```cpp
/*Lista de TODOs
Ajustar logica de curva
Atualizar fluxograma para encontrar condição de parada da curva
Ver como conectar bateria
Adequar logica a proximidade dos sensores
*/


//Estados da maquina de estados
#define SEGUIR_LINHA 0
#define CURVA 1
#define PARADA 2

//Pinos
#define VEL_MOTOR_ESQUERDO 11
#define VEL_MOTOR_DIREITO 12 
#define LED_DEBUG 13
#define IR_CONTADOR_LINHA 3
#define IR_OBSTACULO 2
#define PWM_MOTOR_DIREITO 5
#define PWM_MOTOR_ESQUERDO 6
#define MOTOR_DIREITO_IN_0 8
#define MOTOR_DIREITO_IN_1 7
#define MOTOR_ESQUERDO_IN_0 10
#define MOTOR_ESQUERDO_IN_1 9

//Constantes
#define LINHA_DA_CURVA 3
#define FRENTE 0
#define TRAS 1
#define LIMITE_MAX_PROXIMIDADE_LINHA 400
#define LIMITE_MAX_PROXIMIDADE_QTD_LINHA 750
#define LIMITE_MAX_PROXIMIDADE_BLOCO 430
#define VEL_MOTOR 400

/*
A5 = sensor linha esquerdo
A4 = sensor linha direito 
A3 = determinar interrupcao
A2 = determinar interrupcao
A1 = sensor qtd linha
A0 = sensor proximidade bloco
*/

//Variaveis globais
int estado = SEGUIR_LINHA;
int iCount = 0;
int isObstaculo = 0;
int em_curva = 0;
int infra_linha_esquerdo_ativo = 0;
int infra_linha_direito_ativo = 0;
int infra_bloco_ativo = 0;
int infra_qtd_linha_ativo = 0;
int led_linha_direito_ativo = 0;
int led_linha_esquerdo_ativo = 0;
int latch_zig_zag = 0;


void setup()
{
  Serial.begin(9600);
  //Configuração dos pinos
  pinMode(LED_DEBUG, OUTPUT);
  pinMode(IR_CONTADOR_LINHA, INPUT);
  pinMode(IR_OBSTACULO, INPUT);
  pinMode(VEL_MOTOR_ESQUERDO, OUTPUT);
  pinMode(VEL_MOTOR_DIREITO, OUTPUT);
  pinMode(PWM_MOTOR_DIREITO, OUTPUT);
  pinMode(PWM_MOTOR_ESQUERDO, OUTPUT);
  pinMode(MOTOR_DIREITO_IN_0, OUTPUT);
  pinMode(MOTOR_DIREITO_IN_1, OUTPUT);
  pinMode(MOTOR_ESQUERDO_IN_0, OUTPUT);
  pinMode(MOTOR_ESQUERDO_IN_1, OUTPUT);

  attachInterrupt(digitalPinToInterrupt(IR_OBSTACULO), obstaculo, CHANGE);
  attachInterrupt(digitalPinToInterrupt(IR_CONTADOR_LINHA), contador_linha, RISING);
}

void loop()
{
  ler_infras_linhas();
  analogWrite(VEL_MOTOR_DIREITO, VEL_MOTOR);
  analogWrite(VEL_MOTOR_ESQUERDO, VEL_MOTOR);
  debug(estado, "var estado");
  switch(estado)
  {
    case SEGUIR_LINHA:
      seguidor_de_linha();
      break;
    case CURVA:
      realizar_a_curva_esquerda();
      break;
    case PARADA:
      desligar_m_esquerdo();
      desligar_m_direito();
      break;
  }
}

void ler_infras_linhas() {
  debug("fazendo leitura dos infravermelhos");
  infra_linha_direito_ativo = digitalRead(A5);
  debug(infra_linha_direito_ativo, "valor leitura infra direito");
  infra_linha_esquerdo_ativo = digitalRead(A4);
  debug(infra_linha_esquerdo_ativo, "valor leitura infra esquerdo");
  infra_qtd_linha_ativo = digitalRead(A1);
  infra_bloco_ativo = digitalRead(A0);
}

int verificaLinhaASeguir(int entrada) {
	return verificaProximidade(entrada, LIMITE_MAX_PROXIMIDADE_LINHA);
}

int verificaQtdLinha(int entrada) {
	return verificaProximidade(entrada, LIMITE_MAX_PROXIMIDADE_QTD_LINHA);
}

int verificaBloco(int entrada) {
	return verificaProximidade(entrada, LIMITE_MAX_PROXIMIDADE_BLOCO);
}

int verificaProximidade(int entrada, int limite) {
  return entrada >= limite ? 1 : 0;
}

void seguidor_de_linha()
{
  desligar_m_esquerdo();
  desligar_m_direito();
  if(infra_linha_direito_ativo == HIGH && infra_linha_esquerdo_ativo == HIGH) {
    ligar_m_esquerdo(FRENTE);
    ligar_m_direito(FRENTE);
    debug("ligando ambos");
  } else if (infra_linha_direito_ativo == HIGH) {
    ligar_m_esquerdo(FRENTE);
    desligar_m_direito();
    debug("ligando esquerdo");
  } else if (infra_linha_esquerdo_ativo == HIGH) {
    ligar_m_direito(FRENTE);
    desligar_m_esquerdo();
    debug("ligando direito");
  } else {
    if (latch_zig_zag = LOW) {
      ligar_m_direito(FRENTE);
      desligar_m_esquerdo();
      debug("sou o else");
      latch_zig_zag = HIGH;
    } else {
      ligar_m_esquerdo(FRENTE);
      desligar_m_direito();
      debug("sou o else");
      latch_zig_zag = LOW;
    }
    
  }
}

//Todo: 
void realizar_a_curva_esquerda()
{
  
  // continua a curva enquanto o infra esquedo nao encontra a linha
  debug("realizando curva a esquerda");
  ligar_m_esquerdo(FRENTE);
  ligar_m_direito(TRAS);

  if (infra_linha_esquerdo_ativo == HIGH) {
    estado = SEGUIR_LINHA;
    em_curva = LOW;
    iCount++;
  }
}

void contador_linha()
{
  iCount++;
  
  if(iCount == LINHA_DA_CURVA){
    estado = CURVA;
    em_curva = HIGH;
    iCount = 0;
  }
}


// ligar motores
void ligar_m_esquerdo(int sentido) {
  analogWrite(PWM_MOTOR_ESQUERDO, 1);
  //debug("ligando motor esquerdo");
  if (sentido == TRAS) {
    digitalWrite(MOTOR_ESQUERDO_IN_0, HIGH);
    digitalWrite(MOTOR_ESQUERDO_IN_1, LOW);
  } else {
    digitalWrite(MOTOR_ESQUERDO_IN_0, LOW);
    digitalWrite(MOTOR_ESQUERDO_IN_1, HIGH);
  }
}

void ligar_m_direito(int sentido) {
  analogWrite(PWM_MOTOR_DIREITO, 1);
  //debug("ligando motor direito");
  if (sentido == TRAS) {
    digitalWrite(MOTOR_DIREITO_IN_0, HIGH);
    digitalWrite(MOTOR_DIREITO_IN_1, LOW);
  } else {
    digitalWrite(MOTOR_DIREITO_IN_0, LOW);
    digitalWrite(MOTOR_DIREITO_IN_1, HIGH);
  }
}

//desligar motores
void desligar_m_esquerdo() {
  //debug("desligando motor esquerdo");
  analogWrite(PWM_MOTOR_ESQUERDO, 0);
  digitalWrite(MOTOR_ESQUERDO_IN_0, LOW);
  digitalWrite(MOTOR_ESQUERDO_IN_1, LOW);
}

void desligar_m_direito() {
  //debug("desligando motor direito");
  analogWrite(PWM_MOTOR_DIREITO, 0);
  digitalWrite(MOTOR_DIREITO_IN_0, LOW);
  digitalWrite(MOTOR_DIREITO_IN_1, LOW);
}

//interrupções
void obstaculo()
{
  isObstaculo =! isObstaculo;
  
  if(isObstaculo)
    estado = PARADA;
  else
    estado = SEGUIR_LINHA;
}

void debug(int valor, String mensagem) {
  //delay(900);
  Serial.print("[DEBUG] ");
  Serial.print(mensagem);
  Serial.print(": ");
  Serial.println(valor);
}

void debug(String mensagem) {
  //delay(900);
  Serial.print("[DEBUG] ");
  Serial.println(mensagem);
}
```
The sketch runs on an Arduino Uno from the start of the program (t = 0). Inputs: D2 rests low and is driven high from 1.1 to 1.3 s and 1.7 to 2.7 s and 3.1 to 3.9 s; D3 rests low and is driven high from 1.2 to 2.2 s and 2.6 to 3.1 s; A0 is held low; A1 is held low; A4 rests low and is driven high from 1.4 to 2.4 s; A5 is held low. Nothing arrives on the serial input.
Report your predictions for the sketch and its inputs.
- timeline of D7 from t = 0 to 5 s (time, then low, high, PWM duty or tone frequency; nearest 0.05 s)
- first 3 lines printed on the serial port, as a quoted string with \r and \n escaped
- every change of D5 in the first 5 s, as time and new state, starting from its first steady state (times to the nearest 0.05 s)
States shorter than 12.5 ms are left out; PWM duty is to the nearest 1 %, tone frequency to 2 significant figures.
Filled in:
0 s low; 1.6 s high; 1.8 s low
"[DEBUG] fazendo leitura dos infravermelhos\r\n[DEBUG] valor leitura infra direito: 0\r\n[DEBUG] valor leitura infra esquerdo: 0\r\n"
0 s low; 1.6 s PWM 1 %; 1.8 s low
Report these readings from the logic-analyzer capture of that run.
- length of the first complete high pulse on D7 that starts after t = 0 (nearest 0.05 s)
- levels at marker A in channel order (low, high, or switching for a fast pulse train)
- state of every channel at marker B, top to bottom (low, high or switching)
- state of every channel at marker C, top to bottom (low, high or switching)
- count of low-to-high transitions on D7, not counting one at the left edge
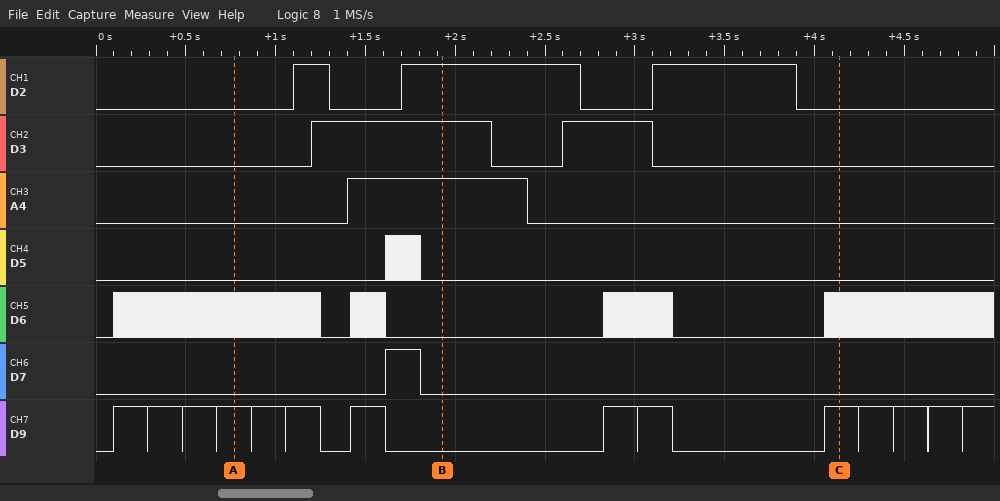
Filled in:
0.20 s
D2 low, D3 low, A4 low, D5 low, D6 switching, D7 low, D9 high
D2 high, D3 high, A4 high, D5 low, D6 low, D7 low, D9 low
D2 low, D3 low, A4 low, D5 low, D6 switching, D7 low, D9 high
1
